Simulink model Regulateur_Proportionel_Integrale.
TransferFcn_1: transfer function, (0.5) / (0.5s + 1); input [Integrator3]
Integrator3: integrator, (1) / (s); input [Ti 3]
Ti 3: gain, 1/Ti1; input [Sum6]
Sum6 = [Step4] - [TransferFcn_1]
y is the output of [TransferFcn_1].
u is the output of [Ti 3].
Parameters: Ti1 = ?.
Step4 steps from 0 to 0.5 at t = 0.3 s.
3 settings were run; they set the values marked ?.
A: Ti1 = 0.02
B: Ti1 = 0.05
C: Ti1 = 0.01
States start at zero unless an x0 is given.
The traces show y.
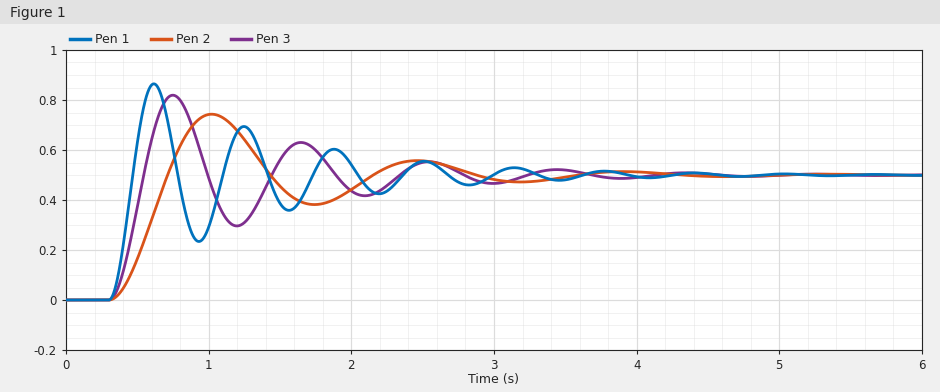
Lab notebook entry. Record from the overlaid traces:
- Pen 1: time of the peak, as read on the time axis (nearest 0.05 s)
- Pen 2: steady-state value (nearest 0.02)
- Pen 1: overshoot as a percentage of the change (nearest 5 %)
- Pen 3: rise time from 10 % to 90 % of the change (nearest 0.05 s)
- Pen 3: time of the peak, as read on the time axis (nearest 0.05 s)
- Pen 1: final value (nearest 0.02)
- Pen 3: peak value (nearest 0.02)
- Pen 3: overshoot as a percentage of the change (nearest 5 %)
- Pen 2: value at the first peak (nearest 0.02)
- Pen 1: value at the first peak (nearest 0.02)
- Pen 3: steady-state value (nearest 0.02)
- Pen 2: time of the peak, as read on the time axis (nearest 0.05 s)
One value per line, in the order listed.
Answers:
0.60 s
0.50
75 %
0.15 s
0.75 s
0.50
0.82
65 %
0.74
0.86
0.50
1.00 s
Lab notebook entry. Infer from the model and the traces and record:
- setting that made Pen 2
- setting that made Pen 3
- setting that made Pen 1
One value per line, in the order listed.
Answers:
B
A
C
